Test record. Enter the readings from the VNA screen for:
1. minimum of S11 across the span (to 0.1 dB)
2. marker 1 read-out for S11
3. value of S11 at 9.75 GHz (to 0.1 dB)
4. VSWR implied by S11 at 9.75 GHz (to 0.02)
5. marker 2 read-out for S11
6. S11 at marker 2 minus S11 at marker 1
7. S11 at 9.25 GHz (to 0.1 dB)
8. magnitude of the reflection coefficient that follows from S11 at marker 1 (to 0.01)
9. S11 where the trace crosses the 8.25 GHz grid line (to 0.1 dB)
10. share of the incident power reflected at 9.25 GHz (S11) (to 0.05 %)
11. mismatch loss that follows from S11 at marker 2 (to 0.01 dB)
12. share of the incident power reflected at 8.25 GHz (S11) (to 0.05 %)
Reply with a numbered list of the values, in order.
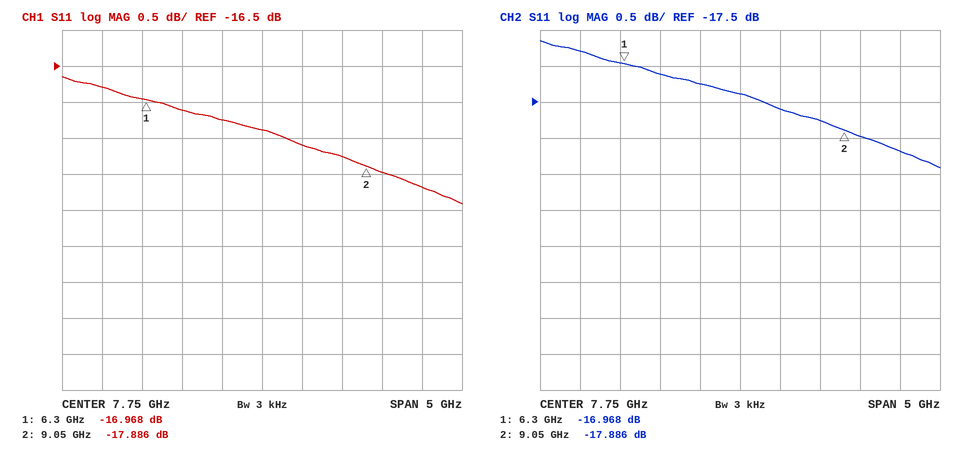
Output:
1. -18.4 dB
2. -16.968 dB
3. -18.2 dB
4. 1.28
5. -17.886 dB
6. -0.918 dB
7. -18.0 dB
8. 0.14
9. -17.6 dB
10. 1.60 %
11. 0.07 dB
12. 1.75 %
